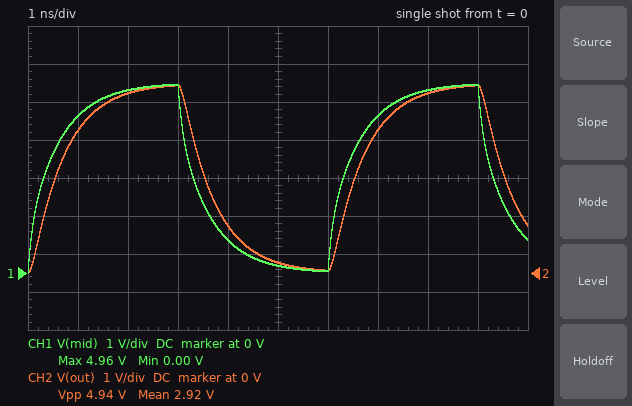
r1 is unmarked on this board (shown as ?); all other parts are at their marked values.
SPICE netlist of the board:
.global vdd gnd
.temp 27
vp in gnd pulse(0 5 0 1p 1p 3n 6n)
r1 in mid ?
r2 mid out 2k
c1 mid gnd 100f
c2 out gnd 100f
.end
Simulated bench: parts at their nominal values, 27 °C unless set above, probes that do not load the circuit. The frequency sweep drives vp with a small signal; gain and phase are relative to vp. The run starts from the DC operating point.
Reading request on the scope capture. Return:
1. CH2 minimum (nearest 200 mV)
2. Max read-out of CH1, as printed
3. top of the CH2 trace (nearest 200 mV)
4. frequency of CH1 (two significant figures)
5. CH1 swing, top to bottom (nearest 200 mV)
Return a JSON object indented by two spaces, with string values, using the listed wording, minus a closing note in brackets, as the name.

{
  "CH2 minimum": "0 V",
  "Max read-out of CH1, as printed": "4.96 V",
  "top of the CH2 trace": "5.0 V",
  "frequency of CH1": "170 MHz",
  "CH1 swing, top to bottom": "5.0 V"
}
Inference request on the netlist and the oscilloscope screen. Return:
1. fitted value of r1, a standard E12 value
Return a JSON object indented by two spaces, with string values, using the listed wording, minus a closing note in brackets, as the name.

{
  "fitted value of r1, a standard E12 value": "2.7 kΩ"
}
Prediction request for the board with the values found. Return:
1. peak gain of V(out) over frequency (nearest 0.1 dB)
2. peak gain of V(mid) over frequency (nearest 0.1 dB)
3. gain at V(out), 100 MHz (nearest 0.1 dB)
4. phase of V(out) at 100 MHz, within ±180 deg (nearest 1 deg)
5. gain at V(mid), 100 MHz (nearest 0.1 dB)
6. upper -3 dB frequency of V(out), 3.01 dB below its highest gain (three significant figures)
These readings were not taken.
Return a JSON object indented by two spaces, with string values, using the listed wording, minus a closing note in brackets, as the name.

{
  "peak gain of V(out) over frequency": "0 dB",
  "peak gain of V(mid) over frequency": "0 dB",
  "gain at V(out), 100 MHz": "-0.7 dB",
  "phase of V(out) at 100 MHz, within ±180 deg": "-25 deg",
  "gain at V(mid), 100 MHz": "-0.6 dB",
  "upper -3 dB frequency of V(out), 3.01 dB below its highest gain": "238 MHz"
}
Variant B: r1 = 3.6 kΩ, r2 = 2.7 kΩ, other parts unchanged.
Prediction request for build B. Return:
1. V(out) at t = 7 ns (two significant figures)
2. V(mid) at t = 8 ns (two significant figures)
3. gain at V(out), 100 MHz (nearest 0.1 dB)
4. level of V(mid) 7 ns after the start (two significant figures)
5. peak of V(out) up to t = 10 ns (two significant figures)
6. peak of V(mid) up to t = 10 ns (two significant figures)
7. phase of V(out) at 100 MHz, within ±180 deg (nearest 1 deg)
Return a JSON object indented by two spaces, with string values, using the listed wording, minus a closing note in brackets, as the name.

{
  "V(out) at t = 7 ns": "3.2 V",
  "V(mid) at t = 8 ns": "4.6 V",
  "gain at V(out), 100 MHz": "-1.2 dB",
  "level of V(mid) 7 ns after the start": "3.8 V",
  "peak of V(out) up to t = 10 ns": "4.8 V",
  "peak of V(mid) up to t = 10 ns": "4.9 V",
  "phase of V(out) at 100 MHz, within ±180 deg": "-33 deg"
}
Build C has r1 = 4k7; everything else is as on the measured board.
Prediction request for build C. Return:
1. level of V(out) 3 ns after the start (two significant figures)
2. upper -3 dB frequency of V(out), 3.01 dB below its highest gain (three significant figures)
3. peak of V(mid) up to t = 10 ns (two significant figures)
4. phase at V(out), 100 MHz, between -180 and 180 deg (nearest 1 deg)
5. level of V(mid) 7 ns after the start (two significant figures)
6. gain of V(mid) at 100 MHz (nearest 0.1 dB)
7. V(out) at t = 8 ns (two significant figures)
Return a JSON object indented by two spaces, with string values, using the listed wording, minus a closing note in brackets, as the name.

{
  "level of V(out) 3 ns after the start": "4.7 V",
  "upper -3 dB frequency of V(out), 3.01 dB below its highest gain": "150 MHz",
  "peak of V(mid) up to t = 10 ns": "4.8 V",
  "phase at V(out), 100 MHz, between -180 and 180 deg": "-37 deg",
  "level of V(mid) 7 ns after the start": "3.4 V",
  "gain of V(mid) at 100 MHz": "-1.5 dB",
  "V(out) at t = 8 ns": "4.2 V"
}
